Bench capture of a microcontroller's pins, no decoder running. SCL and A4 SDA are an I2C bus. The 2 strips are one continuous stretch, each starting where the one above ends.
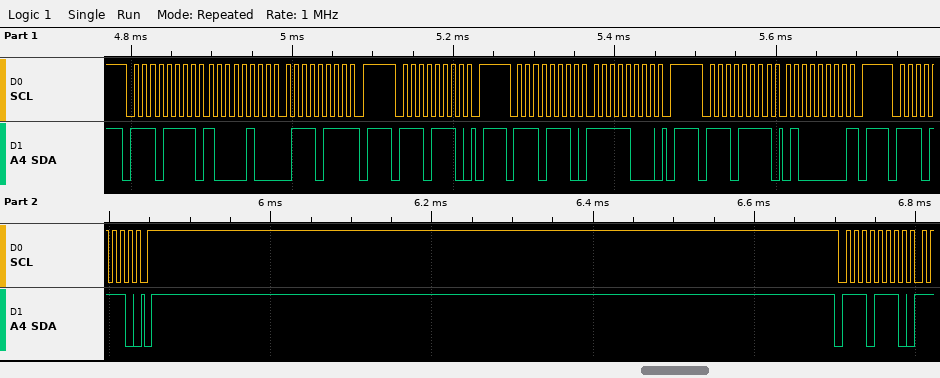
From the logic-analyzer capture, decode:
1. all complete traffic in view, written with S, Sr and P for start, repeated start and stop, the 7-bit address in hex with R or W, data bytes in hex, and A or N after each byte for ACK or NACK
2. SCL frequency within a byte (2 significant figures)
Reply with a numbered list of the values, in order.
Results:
1. S 77R A 84 A 77 N P S 77W A P S 77W A F8 A P S 77R A 40 N P S 77W A P S 77W A
2. 100 kHz
